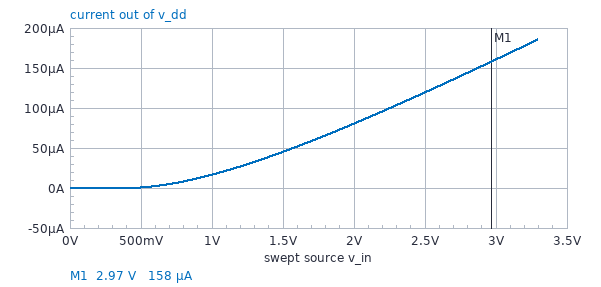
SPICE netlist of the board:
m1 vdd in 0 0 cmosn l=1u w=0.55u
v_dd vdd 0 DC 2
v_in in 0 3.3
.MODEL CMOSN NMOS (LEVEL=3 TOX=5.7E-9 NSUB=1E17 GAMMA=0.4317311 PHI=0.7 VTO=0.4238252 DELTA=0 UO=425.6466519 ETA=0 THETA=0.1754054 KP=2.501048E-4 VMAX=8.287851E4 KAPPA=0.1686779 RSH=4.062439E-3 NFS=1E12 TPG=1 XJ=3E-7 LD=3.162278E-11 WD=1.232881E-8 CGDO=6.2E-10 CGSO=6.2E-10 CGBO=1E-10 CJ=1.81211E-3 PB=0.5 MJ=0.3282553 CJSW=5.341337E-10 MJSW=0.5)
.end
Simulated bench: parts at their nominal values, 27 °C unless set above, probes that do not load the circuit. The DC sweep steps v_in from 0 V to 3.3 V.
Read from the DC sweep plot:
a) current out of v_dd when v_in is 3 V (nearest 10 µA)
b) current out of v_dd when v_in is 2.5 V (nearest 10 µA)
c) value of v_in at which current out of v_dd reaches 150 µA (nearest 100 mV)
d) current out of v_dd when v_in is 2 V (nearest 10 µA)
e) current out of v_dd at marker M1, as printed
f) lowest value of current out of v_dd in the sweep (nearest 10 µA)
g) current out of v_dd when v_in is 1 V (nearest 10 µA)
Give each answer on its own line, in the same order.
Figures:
160 µA
120 µA
2.9 V
80 µA
158 µA
0 A
20 µA
